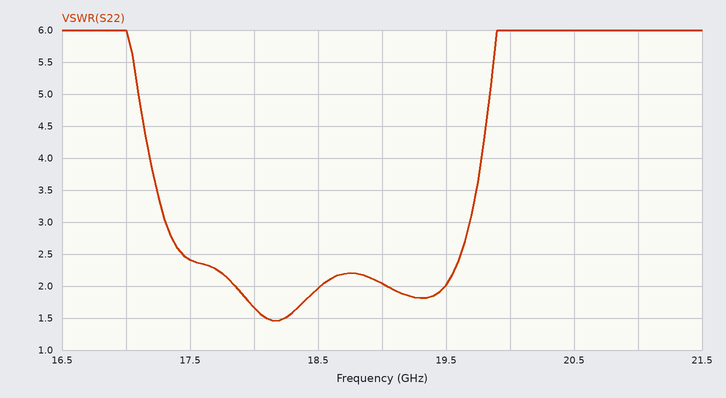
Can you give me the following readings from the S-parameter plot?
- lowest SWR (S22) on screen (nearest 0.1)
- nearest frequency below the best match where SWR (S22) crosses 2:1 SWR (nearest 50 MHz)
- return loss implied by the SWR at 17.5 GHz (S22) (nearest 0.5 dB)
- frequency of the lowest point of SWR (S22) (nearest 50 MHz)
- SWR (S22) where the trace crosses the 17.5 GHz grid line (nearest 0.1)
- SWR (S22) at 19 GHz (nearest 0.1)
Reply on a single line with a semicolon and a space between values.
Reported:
1.5; 17.85 GHz; 7.5 dB; 18.15 GHz; 2.4; 2.0
